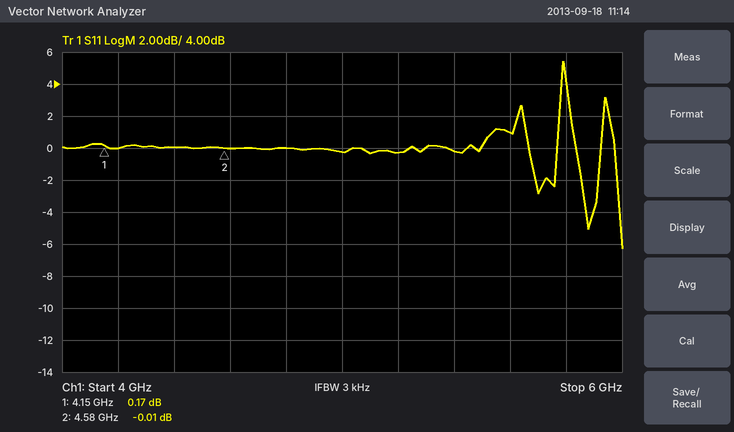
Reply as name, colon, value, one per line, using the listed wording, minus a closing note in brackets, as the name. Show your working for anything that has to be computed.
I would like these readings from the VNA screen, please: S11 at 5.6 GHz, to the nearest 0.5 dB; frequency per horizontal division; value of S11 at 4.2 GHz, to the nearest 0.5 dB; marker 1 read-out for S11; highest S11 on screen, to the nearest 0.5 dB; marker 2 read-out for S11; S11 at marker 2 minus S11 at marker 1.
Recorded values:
S11 at 5.6 GHz, to the nearest 0.5 dB: 1.0 dB
frequency per horizontal division: 200 MHz
value of S11 at 4.2 GHz, to the nearest 0.5 dB: 0.0 dB
marker 1 read-out for S11: 0.17 dB
highest S11 on screen, to the nearest 0.5 dB: 5.5 dB
marker 2 read-out for S11: -0.01 dB
S11 at marker 2 minus S11 at marker 1: -0.01 − (0.17) = -0.18 dB
